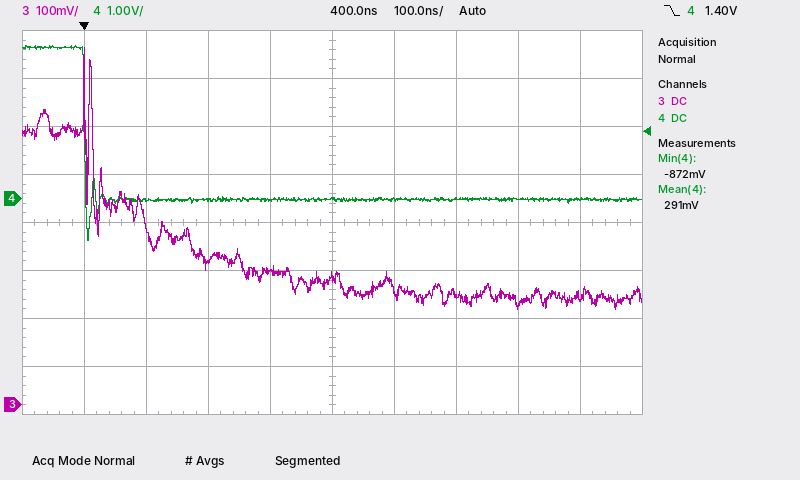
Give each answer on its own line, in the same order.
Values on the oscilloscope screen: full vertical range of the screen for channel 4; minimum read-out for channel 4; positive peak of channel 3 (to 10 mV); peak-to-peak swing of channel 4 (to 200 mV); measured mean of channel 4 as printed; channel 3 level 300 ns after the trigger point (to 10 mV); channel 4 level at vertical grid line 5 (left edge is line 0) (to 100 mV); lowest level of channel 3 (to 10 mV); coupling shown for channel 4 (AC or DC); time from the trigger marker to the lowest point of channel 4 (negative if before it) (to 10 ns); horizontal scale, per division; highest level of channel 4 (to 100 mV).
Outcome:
8 V
-872 mV
740 mV
4.0 V
291 mV
280 mV
0.0 V
200 mV
DC
+10 ns
100 ns
3.2 V
